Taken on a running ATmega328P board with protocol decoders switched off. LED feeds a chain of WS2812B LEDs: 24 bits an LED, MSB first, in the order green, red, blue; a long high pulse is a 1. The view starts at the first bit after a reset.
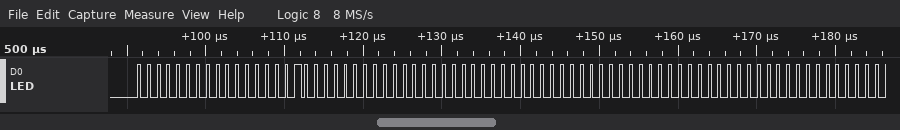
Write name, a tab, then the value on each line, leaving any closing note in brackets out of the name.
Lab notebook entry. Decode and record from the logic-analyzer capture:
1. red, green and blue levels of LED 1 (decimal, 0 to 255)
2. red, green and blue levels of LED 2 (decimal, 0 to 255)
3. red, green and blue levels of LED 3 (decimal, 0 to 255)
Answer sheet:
red, green and blue levels of LED 1	0, 0, 128
red, green and blue levels of LED 2	0, 0, 0
red, green and blue levels of LED 3	0, 0, 0
